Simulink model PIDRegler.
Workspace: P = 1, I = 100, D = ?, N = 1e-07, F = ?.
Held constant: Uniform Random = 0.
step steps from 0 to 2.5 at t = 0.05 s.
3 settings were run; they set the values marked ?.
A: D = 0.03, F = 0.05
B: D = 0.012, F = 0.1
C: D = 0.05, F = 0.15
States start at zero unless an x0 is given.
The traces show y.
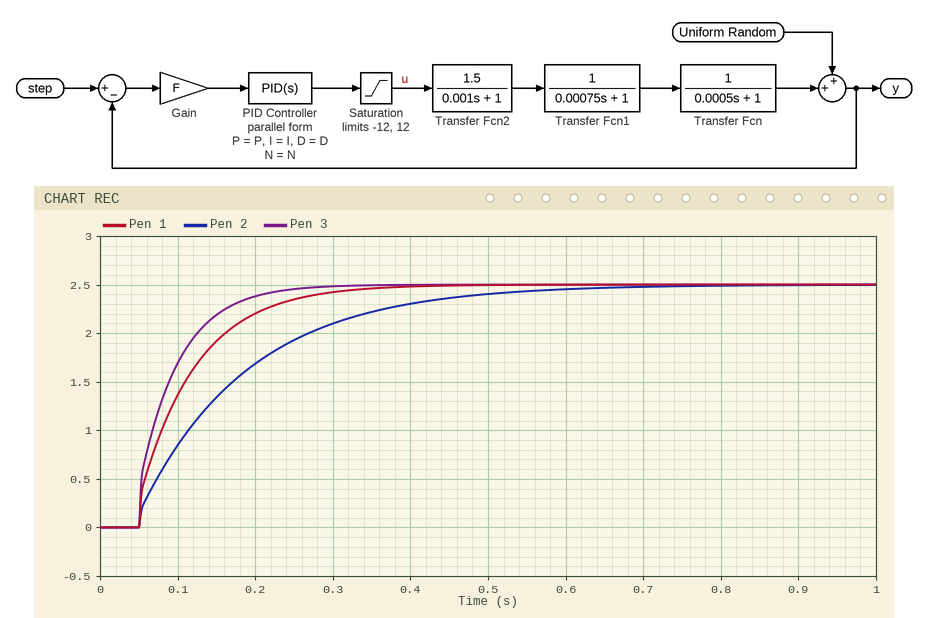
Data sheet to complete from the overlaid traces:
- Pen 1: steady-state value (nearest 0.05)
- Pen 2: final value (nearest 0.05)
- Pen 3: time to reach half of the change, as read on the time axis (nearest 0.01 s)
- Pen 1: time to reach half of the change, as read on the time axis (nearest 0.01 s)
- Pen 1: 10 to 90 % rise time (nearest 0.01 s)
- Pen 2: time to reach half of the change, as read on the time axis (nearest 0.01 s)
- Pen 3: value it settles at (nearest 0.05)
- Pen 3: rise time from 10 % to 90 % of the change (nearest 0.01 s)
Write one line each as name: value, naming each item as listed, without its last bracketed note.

Pen 1: steady-state value: 2.50
Pen 2: final value: 2.50
Pen 3: time to reach half of the change, as read on the time axis: 0.08 s
Pen 1: time to reach half of the change, as read on the time axis: 0.09 s
Pen 1: 10 to 90 % rise time: 0.16 s
Pen 2: time to reach half of the change, as read on the time axis: 0.14 s
Pen 3: value it settles at: 2.50
Pen 3: rise time from 10 % to 90 % of the change: 0.11 s
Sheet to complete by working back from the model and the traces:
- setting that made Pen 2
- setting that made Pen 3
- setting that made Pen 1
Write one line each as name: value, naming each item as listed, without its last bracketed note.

setting that made Pen 2: A
setting that made Pen 3: C
setting that made Pen 1: B
